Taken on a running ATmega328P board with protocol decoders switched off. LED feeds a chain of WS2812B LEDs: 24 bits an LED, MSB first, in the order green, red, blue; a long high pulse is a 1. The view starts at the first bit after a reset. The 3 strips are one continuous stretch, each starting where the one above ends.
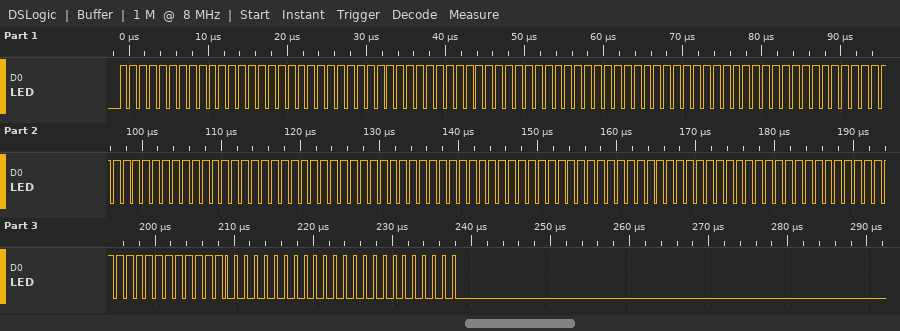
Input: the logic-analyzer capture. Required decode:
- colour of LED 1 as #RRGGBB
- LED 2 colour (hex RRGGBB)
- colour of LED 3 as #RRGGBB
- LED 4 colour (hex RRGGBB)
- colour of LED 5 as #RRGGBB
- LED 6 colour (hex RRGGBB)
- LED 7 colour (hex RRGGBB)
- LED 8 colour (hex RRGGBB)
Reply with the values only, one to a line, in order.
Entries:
#FFFFFF
#FFFFFF
#FFFFFF
#FFFFFF
#FFFFFF
#FFFFFF
#FFFFFF
#000000
